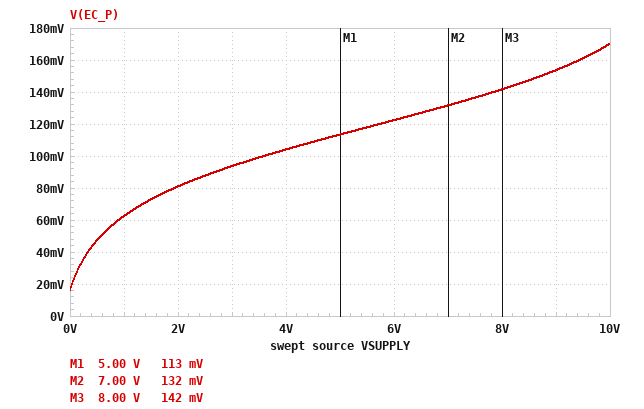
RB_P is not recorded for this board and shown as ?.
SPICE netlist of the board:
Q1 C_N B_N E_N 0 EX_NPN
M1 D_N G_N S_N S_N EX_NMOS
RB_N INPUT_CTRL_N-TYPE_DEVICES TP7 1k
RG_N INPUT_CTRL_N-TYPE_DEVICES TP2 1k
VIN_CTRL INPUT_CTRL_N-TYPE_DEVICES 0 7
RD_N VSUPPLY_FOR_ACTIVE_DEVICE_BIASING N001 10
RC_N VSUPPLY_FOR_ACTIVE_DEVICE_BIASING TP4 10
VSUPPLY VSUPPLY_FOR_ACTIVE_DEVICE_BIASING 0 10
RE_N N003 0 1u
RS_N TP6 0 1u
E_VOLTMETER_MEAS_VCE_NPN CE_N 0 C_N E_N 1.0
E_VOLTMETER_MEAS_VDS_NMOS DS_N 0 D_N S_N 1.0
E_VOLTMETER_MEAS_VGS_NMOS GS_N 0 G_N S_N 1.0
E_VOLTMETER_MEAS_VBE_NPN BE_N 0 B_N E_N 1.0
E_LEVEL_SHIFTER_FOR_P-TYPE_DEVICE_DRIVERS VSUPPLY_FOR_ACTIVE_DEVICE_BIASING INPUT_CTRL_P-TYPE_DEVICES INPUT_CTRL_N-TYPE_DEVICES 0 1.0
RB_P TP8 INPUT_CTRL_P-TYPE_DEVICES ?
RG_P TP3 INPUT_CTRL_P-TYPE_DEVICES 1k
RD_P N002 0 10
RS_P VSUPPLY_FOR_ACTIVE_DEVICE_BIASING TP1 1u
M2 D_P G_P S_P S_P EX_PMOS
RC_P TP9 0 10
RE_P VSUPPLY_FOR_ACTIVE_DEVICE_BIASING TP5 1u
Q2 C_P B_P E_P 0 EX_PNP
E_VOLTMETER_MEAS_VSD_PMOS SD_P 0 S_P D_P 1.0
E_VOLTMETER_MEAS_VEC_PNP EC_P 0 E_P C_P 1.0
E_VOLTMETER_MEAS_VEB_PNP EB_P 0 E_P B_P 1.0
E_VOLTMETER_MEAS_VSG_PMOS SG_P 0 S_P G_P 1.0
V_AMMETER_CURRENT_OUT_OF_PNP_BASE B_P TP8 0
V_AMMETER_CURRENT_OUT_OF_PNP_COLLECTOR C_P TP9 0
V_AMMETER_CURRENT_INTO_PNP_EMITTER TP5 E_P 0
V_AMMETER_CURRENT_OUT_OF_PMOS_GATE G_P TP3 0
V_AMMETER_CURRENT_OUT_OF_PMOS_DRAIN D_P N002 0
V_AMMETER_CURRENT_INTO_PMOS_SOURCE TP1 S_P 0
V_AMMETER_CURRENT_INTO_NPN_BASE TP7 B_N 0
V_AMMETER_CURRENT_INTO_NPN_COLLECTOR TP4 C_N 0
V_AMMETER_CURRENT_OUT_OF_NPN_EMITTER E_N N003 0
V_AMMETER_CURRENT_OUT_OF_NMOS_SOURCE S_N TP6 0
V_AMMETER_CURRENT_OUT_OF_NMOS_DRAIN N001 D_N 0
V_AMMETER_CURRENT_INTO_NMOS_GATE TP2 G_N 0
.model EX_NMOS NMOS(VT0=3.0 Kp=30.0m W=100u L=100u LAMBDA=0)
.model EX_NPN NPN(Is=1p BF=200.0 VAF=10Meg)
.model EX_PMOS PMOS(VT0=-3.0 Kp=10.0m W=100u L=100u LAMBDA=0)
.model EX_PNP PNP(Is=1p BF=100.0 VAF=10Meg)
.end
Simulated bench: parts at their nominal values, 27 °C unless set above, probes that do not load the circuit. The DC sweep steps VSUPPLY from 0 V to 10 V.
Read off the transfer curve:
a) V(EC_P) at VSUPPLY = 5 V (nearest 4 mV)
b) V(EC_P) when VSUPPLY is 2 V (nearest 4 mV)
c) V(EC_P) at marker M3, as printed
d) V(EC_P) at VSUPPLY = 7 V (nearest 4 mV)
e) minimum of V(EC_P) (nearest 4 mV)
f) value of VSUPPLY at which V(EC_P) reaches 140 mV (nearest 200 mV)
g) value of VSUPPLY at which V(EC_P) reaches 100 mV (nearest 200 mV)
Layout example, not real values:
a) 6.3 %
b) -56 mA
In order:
a) 112 mV
b) 80 mV
c) 142 mV
d) 132 mV
e) 16 mV
f) 7.8 V
g) 3.6 V
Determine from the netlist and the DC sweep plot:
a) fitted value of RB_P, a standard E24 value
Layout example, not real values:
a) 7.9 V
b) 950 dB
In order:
a) 560 Ω
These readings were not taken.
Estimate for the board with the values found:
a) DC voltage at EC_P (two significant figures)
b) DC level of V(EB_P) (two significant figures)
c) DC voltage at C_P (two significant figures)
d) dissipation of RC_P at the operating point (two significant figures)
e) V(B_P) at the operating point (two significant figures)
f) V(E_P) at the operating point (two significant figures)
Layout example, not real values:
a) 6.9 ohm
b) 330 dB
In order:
a) 170 mV
b) 710 mV
c) 9.8 V
d) 9.7 W
e) 9.3 V
f) 10 V
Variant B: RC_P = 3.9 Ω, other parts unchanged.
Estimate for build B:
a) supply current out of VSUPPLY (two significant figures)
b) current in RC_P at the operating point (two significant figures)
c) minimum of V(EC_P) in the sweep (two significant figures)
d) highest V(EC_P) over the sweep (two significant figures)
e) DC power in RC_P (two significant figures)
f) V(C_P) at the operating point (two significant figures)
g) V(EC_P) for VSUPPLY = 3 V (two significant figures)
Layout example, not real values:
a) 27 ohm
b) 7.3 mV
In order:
a) 2.4 A
b) 1.1 A
c) 14 mV
d) 5.6 V
e) 4.9 W
f) 4.4 V
g) 140 mV
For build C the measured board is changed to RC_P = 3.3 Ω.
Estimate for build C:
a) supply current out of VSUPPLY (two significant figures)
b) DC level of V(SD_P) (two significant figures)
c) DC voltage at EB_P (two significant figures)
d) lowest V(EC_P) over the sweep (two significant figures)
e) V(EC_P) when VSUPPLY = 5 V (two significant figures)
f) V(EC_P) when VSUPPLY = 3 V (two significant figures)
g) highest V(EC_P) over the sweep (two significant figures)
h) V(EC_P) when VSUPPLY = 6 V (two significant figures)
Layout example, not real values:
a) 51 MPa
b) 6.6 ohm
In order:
a) 2.4 A
b) 9.2 V
c) 720 mV
d) 13 mV
e) 1.3 V
f) 150 mV
g) 6.3 V
h) 2.3 V
